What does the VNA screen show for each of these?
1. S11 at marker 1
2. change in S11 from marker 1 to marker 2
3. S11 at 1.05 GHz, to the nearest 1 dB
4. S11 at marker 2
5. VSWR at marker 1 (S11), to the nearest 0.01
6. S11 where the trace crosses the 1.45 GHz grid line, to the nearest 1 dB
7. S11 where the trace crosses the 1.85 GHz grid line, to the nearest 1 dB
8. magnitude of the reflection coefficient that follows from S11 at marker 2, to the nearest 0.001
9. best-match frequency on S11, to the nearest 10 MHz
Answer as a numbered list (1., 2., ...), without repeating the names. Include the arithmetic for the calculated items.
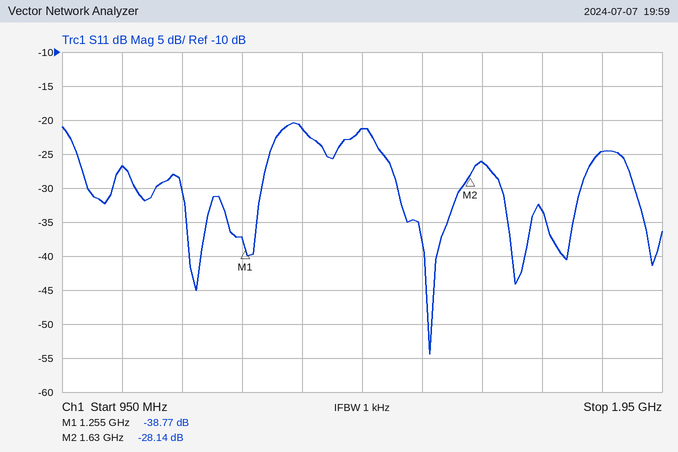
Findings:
1. -38.77 dB
2. -28.14 − (-38.77) = 10.63 dB
3. -27 dB
4. -28.14 dB
5. (1 + 0.0115)/(1 − 0.0115) ≈ 1.02
6. -21 dB
7. -25 dB
8. 10^(-28.14/20) ≈ 0.039
9. 1.56 GHz
